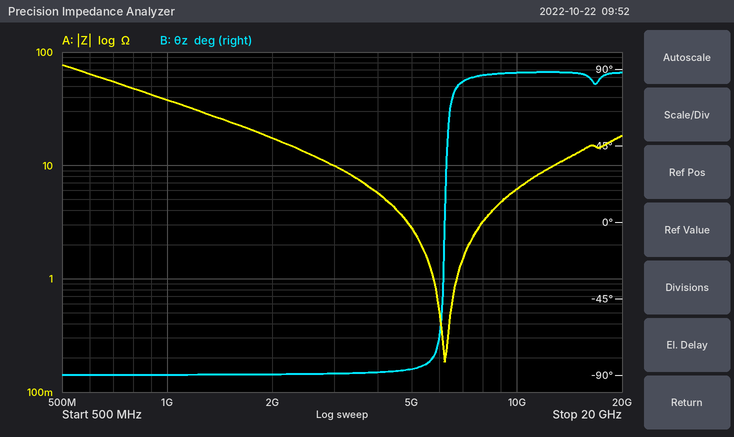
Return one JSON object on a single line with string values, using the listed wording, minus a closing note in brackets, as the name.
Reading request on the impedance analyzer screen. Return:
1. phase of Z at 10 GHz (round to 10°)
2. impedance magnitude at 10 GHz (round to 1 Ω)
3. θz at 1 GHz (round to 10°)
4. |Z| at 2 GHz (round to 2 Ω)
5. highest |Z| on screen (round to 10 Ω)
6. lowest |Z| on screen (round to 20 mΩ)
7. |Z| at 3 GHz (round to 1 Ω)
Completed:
{"phase of Z at 10 GHz": "90°", "impedance magnitude at 10 GHz": "6 Ω", "θz at 1 GHz": "-90°", "|Z| at 2 GHz": "18 Ω", "highest |Z| on screen": "80 Ω", "lowest |Z| on screen": "180 mΩ", "|Z| at 3 GHz": "10 Ω"}
